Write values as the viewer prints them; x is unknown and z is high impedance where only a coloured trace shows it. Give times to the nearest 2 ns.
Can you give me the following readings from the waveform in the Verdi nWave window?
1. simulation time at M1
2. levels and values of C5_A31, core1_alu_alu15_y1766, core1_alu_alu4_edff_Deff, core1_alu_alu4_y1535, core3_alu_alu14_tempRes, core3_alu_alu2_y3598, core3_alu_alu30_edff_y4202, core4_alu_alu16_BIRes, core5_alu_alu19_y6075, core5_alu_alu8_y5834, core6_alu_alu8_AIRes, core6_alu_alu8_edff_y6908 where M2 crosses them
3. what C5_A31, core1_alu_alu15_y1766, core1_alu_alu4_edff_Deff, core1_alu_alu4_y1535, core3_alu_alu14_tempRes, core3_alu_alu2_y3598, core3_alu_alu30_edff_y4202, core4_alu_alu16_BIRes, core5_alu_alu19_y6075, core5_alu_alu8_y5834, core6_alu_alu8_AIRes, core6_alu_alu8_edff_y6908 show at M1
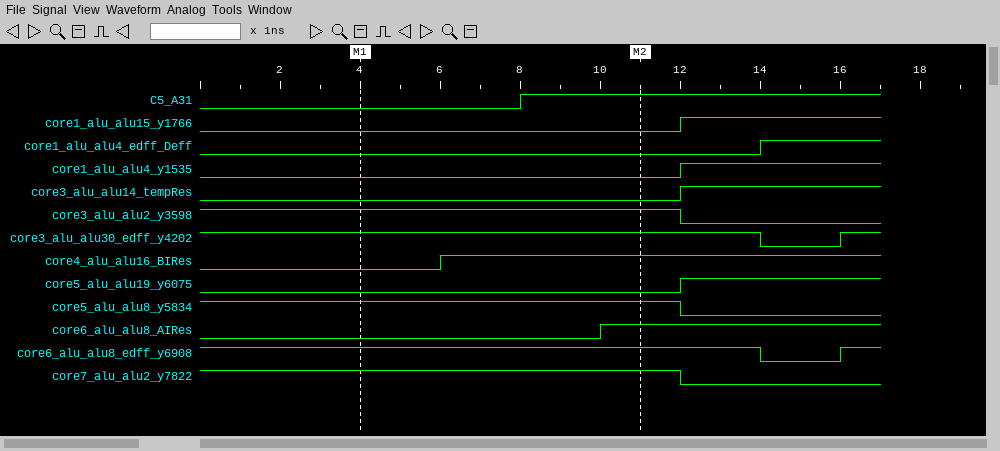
4 ns
C5_A31=1, core1_alu_alu15_y1766=0, core1_alu_alu4_edff_Deff=0, core1_alu_alu4_y1535=0, core3_alu_alu14_tempRes=0, core3_alu_alu2_y3598=1, core3_alu_alu30_edff_y4202=1, core4_alu_alu16_BIRes=1, core5_alu_alu19_y6075=0, core5_alu_alu8_y5834=1, core6_alu_alu8_AIRes=1, core6_alu_alu8_edff_y6908=1
C5_A31=0, core1_alu_alu15_y1766=0, core1_alu_alu4_edff_Deff=0, core1_alu_alu4_y1535=0, core3_alu_alu14_tempRes=0, core3_alu_alu2_y3598=1, core3_alu_alu30_edff_y4202=1, core4_alu_alu16_BIRes=0, core5_alu_alu19_y6075=0, core5_alu_alu8_y5834=1, core6_alu_alu8_AIRes=0, core6_alu_alu8_edff_y6908=1
